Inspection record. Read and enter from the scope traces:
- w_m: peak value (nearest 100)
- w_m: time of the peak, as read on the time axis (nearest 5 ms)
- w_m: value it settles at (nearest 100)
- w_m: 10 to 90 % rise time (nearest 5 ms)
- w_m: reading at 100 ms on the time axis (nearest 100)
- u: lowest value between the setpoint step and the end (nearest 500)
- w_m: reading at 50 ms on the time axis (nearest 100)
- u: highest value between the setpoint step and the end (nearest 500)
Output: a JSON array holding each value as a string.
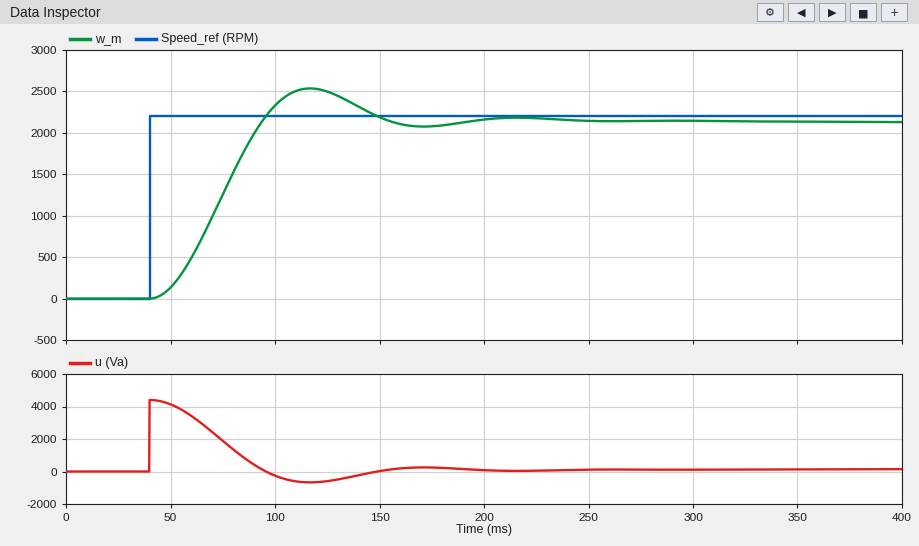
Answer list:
["2500", "115 ms", "2100", "35 ms", "2300", "-500", "100", "4500"]
